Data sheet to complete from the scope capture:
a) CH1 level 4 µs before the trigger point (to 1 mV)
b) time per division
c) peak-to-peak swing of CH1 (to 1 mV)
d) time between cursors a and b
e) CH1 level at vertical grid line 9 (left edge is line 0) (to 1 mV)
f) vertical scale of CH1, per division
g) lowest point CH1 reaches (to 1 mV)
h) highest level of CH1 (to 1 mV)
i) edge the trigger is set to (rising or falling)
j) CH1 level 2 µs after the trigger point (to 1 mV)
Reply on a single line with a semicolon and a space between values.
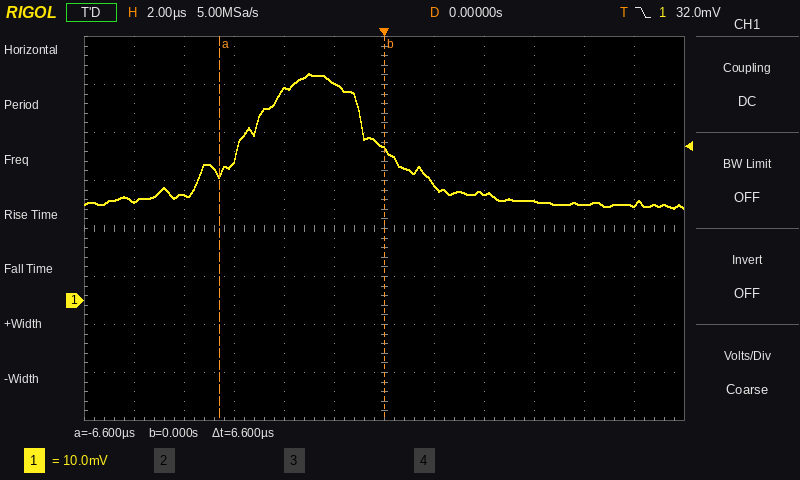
44 mV; 2 µs; 28 mV; 6.6 µs; 21 mV; 10 mV; 19 mV; 47 mV; falling; 24 mV
